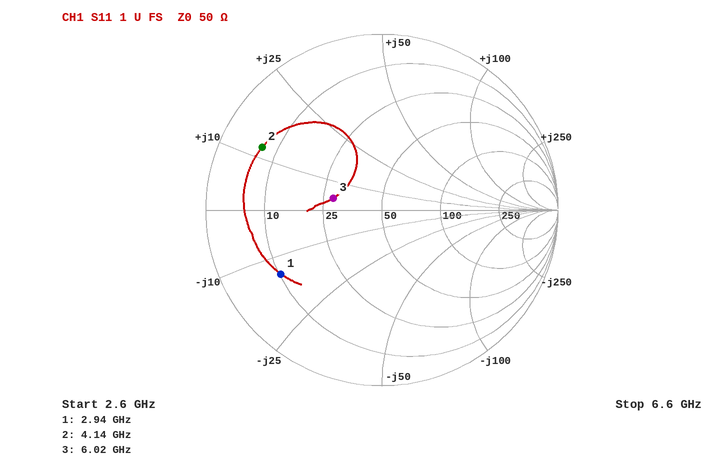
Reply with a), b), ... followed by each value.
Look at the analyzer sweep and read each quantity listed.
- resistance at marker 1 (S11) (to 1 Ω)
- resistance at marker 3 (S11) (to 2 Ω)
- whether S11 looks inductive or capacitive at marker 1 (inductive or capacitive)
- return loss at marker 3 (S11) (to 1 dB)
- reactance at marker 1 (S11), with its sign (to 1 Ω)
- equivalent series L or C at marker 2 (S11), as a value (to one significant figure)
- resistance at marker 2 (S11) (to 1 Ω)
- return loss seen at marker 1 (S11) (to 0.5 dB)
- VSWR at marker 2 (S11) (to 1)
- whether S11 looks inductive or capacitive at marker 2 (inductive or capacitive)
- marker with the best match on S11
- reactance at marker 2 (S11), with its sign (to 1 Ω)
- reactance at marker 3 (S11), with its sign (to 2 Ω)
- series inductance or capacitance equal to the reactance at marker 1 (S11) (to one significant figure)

a) 10 Ω
b) 28 Ω
c) capacitive
d) 11 dB
e) -14 Ω
f) 500 pH
g) 7 Ω
h) 3.5 dB
i) 8
j) inductive
k) marker 3
l) +12 Ω
m) +4 Ω
n) 4 pF
